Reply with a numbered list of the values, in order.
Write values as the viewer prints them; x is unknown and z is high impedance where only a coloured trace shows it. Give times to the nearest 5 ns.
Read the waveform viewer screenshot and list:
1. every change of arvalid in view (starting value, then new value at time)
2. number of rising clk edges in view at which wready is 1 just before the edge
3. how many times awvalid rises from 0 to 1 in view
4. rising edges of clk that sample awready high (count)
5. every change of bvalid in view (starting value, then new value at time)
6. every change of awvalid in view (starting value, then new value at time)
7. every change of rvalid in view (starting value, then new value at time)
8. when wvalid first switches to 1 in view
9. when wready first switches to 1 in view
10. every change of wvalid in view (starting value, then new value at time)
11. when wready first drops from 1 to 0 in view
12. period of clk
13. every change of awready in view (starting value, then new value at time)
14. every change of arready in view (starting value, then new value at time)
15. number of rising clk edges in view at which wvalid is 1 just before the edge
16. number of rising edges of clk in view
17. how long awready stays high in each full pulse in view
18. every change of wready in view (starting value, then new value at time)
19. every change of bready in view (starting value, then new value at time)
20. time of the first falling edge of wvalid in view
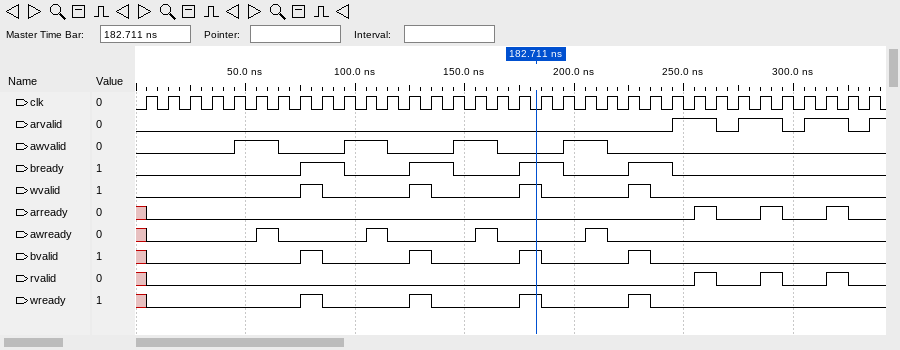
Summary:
1. 0, 1 at 245 ns, 0 at 265 ns, 1 at 275 ns, 0 at 295 ns, 1 at 305 ns, 0 at 325 ns, 1 at 335 ns
2. 4
3. 4
4. 4
5. x, 0 at 5 ns, 1 at 75 ns, 0 at 85 ns, 1 at 125 ns, 0 at 135 ns, 1 at 175 ns, 0 at 185 ns, 1 at 225 ns, 0 at 235 ns
6. 0, 1 at 45 ns, 0 at 65 ns, 1 at 95 ns, 0 at 115 ns, 1 at 145 ns, 0 at 165 ns, 1 at 195 ns, 0 at 215 ns
7. x, 0 at 5 ns, 1 at 255 ns, 0 at 265 ns, 1 at 285 ns, 0 at 295 ns, 1 at 315 ns, 0 at 325 ns
8. 75 ns
9. 75 ns
10. 0, 1 at 75 ns, 0 at 85 ns, 1 at 125 ns, 0 at 135 ns, 1 at 175 ns, 0 at 185 ns, 1 at 225 ns, 0 at 235 ns
11. 85 ns
12. 10 ns
13. x, 0 at 5 ns, 1 at 55 ns, 0 at 65 ns, 1 at 105 ns, 0 at 115 ns, 1 at 155 ns, 0 at 165 ns, 1 at 205 ns, 0 at 215 ns
14. x, 0 at 5 ns, 1 at 255 ns, 0 at 265 ns, 1 at 285 ns, 0 at 295 ns, 1 at 315 ns, 0 at 325 ns
15. 4
16. 34
17. 10 ns, 10 ns, 10 ns, 10 ns
18. x, 0 at 5 ns, 1 at 75 ns, 0 at 85 ns, 1 at 125 ns, 0 at 135 ns, 1 at 175 ns, 0 at 185 ns, 1 at 225 ns, 0 at 235 ns
19. 0, 1 at 75 ns, 0 at 95 ns, 1 at 125 ns, 0 at 145 ns, 1 at 175 ns, 0 at 195 ns, 1 at 225 ns, 0 at 245 ns
20. 85 ns
